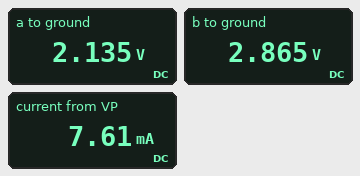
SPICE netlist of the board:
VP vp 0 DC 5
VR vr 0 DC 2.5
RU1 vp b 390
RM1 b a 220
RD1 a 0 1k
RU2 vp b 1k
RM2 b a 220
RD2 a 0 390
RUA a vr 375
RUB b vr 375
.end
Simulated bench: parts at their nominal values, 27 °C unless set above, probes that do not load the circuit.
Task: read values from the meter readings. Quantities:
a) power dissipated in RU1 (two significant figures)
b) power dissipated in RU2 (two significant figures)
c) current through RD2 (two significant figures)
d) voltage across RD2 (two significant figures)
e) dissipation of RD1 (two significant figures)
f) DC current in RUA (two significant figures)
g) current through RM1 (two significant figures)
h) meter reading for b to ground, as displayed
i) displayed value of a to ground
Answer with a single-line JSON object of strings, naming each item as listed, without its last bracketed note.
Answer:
{"power dissipated in RU1": "12 mW", "power dissipated in RU2": "4.6 mW", "current through RD2": "5.5 mA", "voltage across RD2": "2.1 V", "dissipation of RD1": "4.6 mW", "DC current in RUA": "970 µA", "current through RM1": "3.3 mA", "meter reading for b to ground, as displayed": "2.865 V", "displayed value of a to ground": "2.135 V"}
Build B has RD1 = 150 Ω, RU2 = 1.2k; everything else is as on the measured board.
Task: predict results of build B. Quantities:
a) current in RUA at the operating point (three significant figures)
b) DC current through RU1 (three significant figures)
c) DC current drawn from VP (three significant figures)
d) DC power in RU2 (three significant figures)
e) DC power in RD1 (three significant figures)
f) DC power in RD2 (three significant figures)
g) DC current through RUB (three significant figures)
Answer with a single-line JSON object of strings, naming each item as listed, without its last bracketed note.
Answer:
{"current in RUA at the operating point": "3.09 mA", "DC current through RU1": "6.75 mA", "DC current drawn from VP": "8.95 mA", "DC power in RU2": "5.78 mW", "DC power in RD1": "12.0 mW", "DC power in RD2": "4.62 mW", "DC current through RUB": "357 µA"}
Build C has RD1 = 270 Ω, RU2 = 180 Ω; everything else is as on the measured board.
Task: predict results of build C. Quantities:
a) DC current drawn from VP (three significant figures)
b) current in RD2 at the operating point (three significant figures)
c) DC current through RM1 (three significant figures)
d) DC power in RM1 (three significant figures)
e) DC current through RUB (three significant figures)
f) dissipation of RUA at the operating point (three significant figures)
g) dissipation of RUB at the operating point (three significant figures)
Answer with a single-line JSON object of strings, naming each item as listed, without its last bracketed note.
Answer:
{"DC current drawn from VP": "13.7 mA", "current in RD2 at the operating point": "5.23 mA", "DC current through RM1": "5.78 mA", "DC power in RM1": "7.34 mW", "DC current through RUB": "2.16 mA", "dissipation of RUA at the operating point": "565 µW", "dissipation of RUB at the operating point": "1.75 mW"}
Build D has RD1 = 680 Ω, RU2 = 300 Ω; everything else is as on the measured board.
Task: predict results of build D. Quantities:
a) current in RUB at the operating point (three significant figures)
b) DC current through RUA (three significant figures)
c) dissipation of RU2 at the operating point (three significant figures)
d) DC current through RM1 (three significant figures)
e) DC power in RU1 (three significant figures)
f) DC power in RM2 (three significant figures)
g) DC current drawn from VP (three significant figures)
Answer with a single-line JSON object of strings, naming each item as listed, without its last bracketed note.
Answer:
{"current in RUB at the operating point": "1.92 mA", "DC current through RUA": "599 µA", "dissipation of RU2 at the operating point": "10.6 mW", "DC current through RM1": "4.29 mA", "DC power in RU1": "8.13 mW", "DC power in RM2": "4.05 mW", "DC current drawn from VP": "10.5 mA"}
